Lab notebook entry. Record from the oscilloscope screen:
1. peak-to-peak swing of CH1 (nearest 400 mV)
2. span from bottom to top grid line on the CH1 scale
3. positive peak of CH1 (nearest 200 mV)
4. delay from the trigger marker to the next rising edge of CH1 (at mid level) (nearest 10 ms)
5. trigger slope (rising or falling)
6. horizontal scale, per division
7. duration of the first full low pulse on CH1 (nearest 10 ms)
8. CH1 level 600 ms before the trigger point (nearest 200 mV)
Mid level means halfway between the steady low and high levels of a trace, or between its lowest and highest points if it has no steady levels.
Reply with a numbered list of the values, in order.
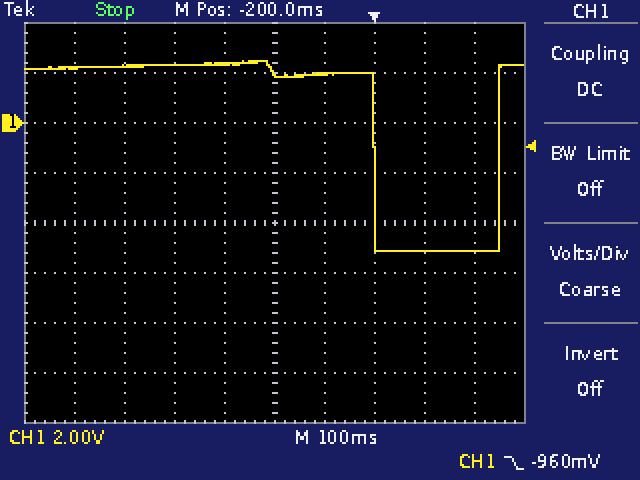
1. 7.6 V
2. 16 V
3. 2.4 V
4. 250 ms
5. falling
6. 100 ms
7. 250 ms
8. 2.2 V
